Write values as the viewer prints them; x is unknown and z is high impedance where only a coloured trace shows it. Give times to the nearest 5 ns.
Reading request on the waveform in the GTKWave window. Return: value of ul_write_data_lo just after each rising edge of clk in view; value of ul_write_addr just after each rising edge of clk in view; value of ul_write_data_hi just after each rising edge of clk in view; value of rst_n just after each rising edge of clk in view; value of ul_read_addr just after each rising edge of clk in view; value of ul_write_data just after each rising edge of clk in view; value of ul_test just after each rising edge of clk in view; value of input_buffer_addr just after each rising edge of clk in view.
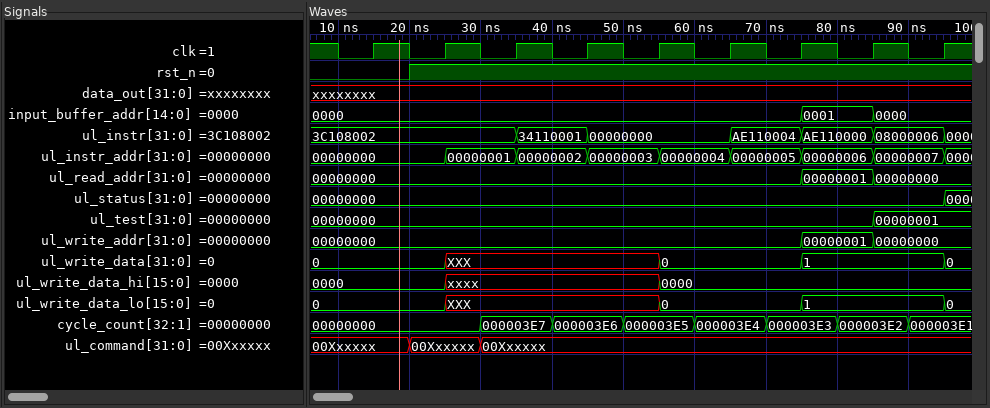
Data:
0, XXX, XXX, XXX, 0, 0, 1, 1, 0
00000000, 00000000, 00000000, 00000000, 00000000, 00000000, 00000001, 00000000, 00000000
0000, xxxx, xxxx, xxxx, 0000, 0000, 0000, 0000, 0000
0 1 1 1 1 1 1 1 1
00000000, 00000000, 00000000, 00000000, 00000000, 00000000, 00000001, 00000000, 00000000
0, XXX, XXX, XXX, 0, 0, 1, 1, 0
00000000, 00000000, 00000000, 00000000, 00000000, 00000000, 00000000, 00000001, 00000001
0000, 0000, 0000, 0000, 0000, 0000, 0001, 0000, 0000
